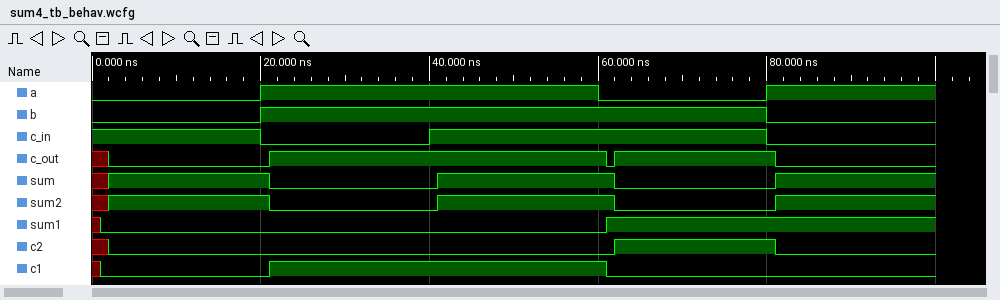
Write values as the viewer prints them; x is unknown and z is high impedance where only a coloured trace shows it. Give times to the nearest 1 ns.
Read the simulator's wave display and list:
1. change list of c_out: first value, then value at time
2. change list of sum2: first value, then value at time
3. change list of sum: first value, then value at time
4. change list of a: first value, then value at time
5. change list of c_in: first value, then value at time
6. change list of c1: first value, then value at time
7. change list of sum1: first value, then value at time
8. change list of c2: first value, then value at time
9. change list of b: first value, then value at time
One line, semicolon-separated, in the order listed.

x, 0 at 2 ns, 1 at 21 ns, 0 at 61 ns, 1 at 62 ns, 0 at 81 ns; x, 1 at 2 ns, 0 at 21 ns, 1 at 41 ns, 0 at 62 ns, 1 at 81 ns; x, 1 at 2 ns, 0 at 21 ns, 1 at 41 ns, 0 at 62 ns, 1 at 81 ns; 0, 1 at 20 ns, 0 at 60 ns, 1 at 80 ns; 1, 0 at 20 ns, 1 at 40 ns, 0 at 80 ns; x, 0 at 1 ns, 1 at 21 ns, 0 at 61 ns; x, 0 at 1 ns, 1 at 61 ns; x, 0 at 2 ns, 1 at 62 ns, 0 at 81 ns; 0, 1 at 20 ns, 0 at 80 ns
